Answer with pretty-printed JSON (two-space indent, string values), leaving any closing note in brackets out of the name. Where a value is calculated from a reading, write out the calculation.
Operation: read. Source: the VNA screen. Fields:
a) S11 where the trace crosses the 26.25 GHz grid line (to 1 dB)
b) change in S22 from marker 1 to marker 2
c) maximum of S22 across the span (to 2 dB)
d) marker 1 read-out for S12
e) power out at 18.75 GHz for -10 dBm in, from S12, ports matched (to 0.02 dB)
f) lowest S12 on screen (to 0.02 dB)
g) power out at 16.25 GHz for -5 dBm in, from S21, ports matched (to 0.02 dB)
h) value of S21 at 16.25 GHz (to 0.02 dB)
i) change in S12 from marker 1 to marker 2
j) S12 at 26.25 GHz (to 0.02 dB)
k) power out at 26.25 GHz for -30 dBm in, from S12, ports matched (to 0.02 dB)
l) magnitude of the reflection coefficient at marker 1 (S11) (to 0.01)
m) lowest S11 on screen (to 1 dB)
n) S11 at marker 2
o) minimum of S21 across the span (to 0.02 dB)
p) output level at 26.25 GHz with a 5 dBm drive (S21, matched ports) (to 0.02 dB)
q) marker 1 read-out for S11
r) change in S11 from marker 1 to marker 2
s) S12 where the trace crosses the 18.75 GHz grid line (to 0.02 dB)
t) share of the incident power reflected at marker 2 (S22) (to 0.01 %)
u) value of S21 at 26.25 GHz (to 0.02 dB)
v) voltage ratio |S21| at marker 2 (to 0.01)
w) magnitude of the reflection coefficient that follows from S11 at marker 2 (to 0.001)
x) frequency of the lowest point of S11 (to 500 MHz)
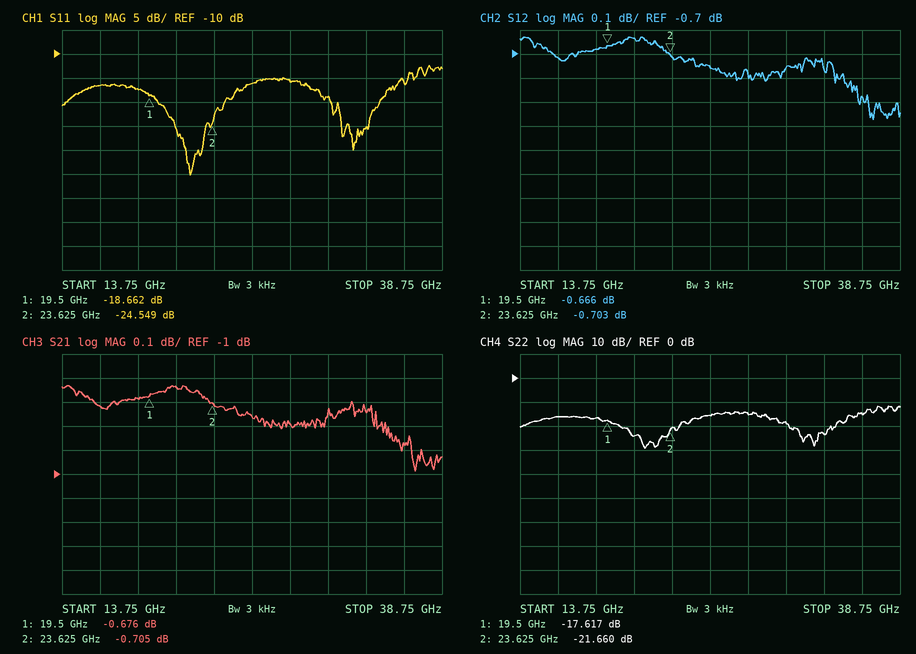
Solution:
{
  "S11 where the trace crosses the 26.25 GHz grid line": "-16 dB",
  "change in S22 from marker 1 to marker 2": "-21.66 − (-17.617) = -4.043 dB",
  "maximum of S22 across the span": "-12 dB",
  "marker 1 read-out for S12": "-0.666 dB",
  "power out at 18.75 GHz for -10 dBm in, from S12, ports matched": "-10 dBm + (-0.68 dB) = -10.68 dBm",
  "lowest S12 on screen": "-0.98 dB",
  "power out at 16.25 GHz for -5 dBm in, from S21, ports matched": "-5 dBm + (-0.72 dB) = -5.72 dBm",
  "value of S21 at 16.25 GHz": "-0.72 dB",
  "change in S12 from marker 1 to marker 2": "-0.703 − (-0.666) = -0.037 dB",
  "S12 at 26.25 GHz": "-0.76 dB",
  "power out at 26.25 GHz for -30 dBm in, from S12, ports matched": "-30 dBm + (-0.76 dB) = -30.76 dBm",
  "magnitude of the reflection coefficient at marker 1 (S11)": "10^(-18.662/20) ≈ 0.12",
  "lowest S11 on screen": "-35 dB",
  "S11 at marker 2": "-24.549 dB",
  "minimum of S21 across the span": "-0.98 dB",
  "output level at 26.25 GHz with a 5 dBm drive (S21, matched ports)": "5 dBm + (-0.76 dB) = 4.24 dBm",
  "marker 1 read-out for S11": "-18.662 dB",
  "change in S11 from marker 1 to marker 2": "-24.549 − (-18.662) = -5.887 dB",
  "S12 where the trace crosses the 18.75 GHz grid line": "-0.68 dB",
  "share of the incident power reflected at marker 2 (S22)": "10^(-21.66/10) ≈ 0.68 %",
  "value of S21 at 26.25 GHz": "-0.76 dB",
  "voltage ratio |S21| at marker 2": "10^(-0.705/20) ≈ 0.92",
  "magnitude of the reflection coefficient that follows from S11 at marker 2": "10^(-24.549/20) ≈ 0.059",
  "frequency of the lowest point of S11": "22.0 GHz"
}
